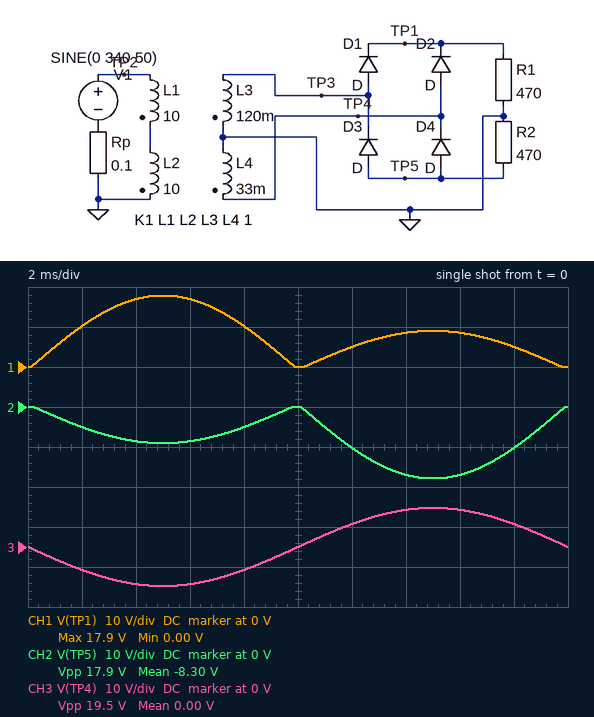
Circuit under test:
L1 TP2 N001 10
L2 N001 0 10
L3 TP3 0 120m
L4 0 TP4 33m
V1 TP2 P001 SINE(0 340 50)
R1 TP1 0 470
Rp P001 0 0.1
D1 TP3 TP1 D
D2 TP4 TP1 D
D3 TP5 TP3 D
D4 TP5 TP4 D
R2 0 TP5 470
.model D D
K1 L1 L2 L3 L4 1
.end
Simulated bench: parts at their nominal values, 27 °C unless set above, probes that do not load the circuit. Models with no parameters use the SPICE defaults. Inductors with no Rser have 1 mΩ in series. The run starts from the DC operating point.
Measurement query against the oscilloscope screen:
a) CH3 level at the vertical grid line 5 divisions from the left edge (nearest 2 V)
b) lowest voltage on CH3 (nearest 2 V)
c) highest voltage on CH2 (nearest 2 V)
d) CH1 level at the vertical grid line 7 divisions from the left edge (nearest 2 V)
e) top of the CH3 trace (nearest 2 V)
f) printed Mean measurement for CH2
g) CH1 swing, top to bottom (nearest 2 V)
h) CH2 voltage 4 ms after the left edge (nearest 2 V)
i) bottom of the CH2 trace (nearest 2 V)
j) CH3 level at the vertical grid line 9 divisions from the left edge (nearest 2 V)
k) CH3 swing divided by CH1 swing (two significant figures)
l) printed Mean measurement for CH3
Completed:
0 V
-10 V
0 V
8 V
10 V
-8.30 V
18 V
-8 V
-18 V
6 V
1.1
0.00 V
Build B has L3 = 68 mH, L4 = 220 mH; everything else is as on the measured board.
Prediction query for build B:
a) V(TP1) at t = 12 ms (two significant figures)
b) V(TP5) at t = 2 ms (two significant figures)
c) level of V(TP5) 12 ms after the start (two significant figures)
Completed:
14 V
-14 V
-7.5 V
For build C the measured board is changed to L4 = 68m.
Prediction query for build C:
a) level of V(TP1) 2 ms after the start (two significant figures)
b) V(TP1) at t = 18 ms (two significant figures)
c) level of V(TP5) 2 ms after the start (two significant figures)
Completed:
10 V
7.5 V
-7.5 V
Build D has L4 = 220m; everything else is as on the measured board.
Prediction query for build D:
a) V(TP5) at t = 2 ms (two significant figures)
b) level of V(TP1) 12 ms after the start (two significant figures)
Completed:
-14 V
14 V
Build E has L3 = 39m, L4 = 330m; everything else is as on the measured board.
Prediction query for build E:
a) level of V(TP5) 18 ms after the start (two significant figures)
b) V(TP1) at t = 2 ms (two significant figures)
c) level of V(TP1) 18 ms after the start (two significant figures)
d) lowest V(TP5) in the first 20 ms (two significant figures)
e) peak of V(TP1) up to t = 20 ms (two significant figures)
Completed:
-5.5 V
5.5 V
17 V
-30 V
30 V
